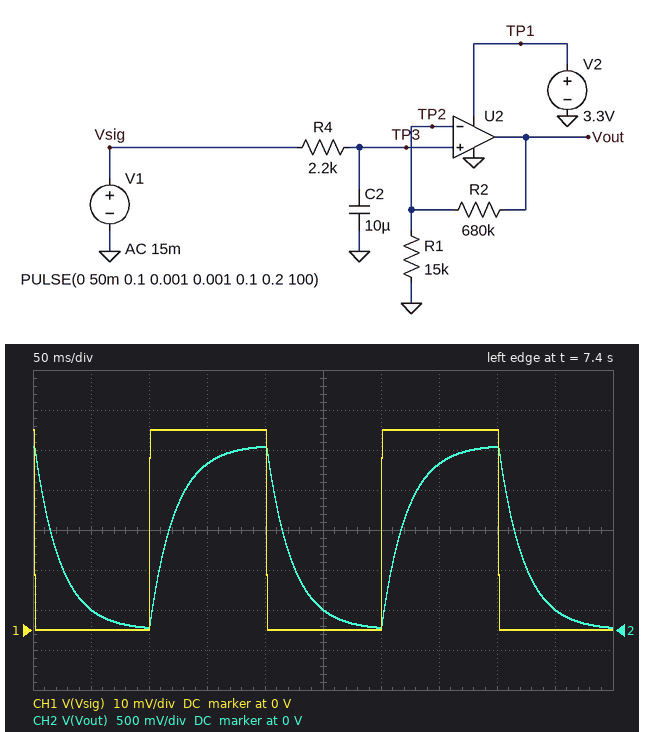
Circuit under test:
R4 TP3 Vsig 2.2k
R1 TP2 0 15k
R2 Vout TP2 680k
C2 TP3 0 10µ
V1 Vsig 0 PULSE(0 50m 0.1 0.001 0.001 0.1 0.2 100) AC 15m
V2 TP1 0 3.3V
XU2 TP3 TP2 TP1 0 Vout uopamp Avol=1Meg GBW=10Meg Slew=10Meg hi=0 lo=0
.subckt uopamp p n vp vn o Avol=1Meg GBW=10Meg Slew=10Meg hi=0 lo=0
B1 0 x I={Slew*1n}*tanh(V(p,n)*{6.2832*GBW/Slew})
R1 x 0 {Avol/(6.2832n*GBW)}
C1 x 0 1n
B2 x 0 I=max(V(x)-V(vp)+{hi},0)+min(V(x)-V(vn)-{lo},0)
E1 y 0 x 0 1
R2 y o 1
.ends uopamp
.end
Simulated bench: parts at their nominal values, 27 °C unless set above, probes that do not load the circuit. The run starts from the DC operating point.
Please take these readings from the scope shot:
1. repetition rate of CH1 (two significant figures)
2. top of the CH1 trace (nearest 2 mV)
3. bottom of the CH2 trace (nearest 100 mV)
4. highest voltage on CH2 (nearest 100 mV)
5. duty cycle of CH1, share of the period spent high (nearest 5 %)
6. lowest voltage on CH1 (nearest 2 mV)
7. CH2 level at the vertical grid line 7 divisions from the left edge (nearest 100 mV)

5.0 Hz
50 mV
0 V
2.3 V
50 %
0 V
2.1 V
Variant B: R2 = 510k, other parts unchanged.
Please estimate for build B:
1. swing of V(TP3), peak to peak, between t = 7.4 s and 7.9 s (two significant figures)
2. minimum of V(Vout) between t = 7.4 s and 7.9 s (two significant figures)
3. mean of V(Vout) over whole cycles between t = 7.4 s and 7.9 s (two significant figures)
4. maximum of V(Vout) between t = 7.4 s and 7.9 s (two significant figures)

49 mV
20 mV
880 mV
1.7 V
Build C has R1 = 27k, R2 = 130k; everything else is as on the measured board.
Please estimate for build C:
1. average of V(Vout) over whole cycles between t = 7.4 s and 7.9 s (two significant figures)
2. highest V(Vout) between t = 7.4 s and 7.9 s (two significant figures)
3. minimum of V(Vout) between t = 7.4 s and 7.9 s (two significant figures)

150 mV
290 mV
3.3 mV
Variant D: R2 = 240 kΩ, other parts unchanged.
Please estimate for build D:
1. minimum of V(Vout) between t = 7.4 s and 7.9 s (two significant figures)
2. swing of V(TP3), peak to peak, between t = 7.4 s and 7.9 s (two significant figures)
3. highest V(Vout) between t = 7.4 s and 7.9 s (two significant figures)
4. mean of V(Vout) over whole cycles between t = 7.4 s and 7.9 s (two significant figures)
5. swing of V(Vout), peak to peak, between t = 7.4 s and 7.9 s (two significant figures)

9.6 mV
49 mV
840 mV
430 mV
830 mV
